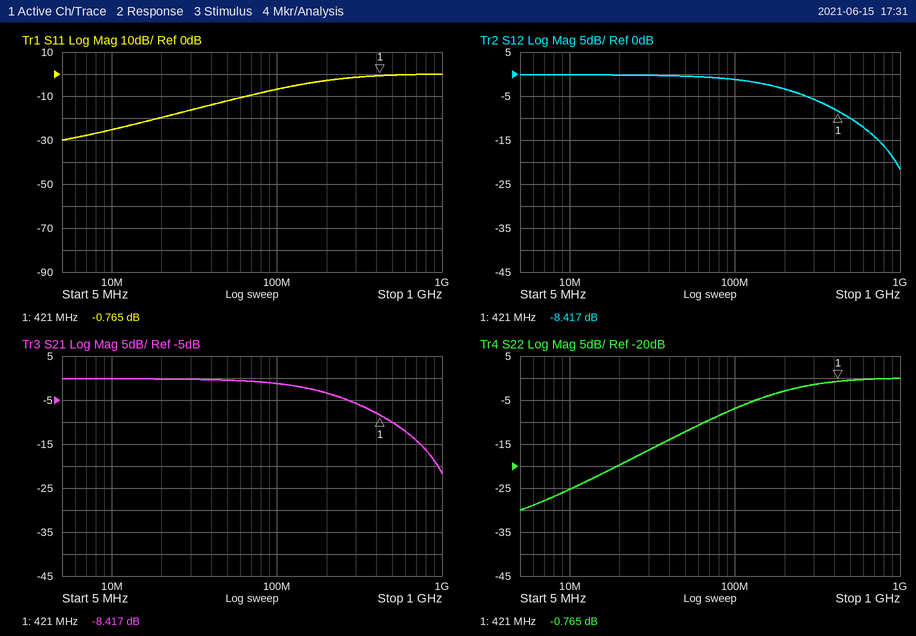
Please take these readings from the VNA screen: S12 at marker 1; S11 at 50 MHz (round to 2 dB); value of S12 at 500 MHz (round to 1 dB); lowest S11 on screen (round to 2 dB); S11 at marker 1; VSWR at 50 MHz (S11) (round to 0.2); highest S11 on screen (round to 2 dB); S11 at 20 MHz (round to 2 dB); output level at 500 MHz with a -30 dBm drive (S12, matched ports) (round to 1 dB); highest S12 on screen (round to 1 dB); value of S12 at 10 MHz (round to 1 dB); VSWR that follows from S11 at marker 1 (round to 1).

-8.417 dB
-12 dB
-10 dB
-30 dB
-0.765 dB
1.6
0 dB
-20 dB
-40 dBm
0 dB
0 dB
23
